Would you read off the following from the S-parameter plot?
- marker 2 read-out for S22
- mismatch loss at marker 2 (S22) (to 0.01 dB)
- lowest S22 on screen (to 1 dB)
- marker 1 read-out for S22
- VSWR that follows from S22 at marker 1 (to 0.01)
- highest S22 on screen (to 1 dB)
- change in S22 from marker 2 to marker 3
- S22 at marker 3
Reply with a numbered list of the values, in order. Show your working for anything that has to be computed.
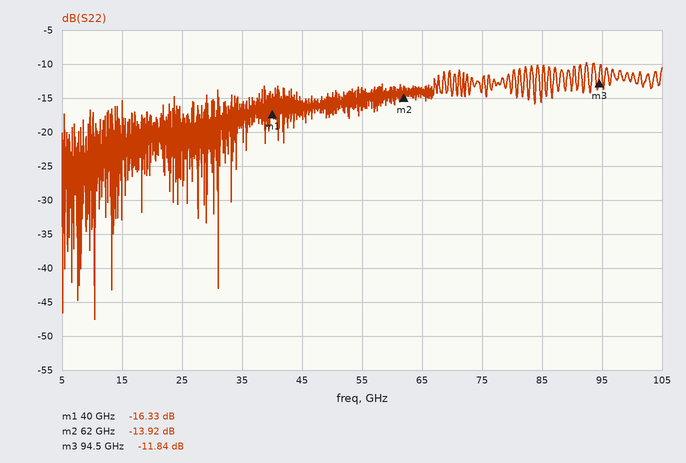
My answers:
1. -13.92 dB
2. −10 log10(1 − 10^(-13.92/10)) ≈ 0.18 dB
3. -48 dB
4. -16.33 dB
5. (1 + 0.1526)/(1 − 0.1526) ≈ 1.36
6. -10 dB
7. -11.84 − (-13.92) = 2.08 dB
8. -11.84 dB
